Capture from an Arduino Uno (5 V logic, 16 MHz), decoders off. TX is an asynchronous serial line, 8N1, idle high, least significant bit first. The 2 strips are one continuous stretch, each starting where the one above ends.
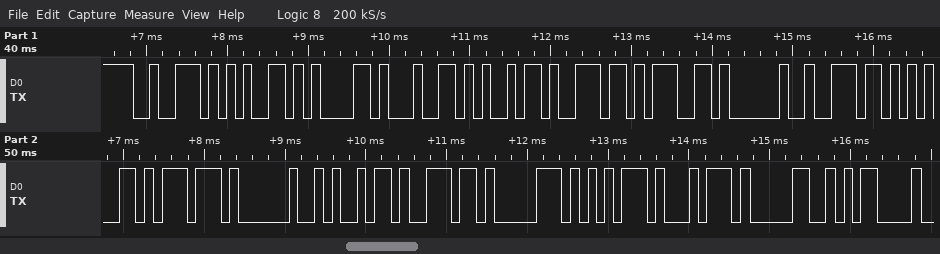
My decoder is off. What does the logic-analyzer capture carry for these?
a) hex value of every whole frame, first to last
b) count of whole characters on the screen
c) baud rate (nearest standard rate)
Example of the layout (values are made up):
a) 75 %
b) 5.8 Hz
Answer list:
a) 72 65 61 64 69 6E 67 20 6E 65 77 20 69 6E 70 75 74 30 0D
b) 19
c) 9600 baud
